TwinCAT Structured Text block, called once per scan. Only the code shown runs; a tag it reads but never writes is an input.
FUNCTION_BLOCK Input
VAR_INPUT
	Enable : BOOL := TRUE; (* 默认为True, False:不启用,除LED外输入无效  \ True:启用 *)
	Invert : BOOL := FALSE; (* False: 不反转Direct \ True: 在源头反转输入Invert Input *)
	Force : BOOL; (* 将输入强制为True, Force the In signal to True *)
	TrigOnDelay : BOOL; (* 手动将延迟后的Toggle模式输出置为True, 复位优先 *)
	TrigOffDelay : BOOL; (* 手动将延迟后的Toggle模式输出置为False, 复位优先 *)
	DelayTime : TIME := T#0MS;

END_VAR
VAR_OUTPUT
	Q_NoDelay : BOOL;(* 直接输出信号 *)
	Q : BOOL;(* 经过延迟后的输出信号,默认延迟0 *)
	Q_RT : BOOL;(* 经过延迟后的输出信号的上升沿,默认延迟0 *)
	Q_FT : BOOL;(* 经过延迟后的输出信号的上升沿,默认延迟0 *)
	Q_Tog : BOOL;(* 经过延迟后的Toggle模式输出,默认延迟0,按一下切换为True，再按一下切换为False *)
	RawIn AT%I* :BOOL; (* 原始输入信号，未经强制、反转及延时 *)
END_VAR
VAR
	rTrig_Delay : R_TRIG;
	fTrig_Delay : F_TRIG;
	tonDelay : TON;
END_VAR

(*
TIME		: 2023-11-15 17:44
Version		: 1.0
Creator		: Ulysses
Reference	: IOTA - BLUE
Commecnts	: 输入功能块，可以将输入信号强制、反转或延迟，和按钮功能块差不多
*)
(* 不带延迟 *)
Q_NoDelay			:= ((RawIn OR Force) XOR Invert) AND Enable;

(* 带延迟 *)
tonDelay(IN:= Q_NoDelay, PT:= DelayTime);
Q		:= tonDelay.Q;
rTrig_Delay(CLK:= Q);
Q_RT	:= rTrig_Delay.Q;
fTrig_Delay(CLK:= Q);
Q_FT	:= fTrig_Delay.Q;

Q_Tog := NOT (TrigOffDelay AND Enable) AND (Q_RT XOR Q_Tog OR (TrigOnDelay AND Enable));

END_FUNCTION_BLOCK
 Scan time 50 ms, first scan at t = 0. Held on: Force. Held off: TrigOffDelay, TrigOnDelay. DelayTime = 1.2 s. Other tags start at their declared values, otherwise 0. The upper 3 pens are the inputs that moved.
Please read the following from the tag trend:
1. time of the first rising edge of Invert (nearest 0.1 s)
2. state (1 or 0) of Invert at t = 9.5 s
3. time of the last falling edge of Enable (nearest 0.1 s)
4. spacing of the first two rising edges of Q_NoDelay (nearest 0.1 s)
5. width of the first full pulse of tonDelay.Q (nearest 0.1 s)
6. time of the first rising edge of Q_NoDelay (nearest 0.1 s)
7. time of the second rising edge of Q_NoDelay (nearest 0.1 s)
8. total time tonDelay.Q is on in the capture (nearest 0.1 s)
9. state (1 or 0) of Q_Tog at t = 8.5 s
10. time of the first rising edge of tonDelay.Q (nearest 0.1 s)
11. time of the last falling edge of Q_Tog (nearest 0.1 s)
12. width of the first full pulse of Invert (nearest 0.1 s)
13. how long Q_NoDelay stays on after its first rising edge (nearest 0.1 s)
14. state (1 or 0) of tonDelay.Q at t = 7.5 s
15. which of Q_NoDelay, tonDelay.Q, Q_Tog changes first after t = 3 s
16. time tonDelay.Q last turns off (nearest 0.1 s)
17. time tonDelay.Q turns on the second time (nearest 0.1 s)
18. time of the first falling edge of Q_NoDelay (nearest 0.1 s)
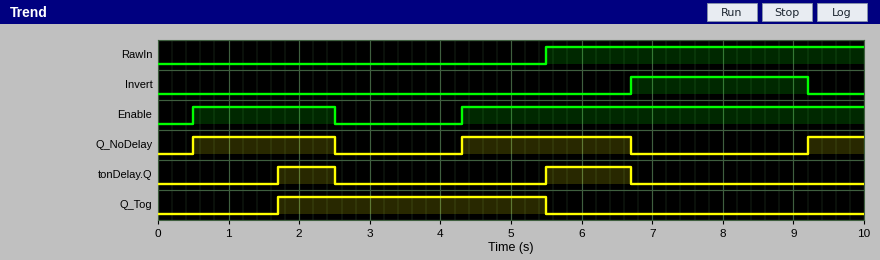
6.7 s
0
2.5 s
3.8 s
0.8 s
0.5 s
4.3 s
2.0 s
0
1.7 s
5.5 s
2.5 s
2.0 s
0
Q_NoDelay
6.7 s
5.5 s
2.5 s
